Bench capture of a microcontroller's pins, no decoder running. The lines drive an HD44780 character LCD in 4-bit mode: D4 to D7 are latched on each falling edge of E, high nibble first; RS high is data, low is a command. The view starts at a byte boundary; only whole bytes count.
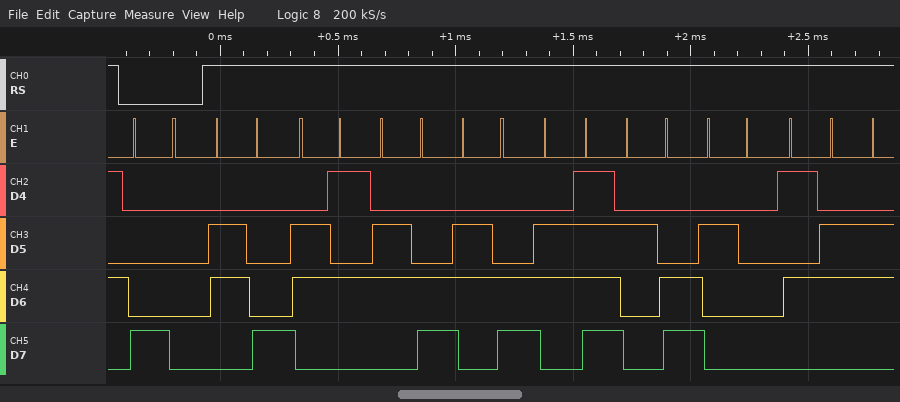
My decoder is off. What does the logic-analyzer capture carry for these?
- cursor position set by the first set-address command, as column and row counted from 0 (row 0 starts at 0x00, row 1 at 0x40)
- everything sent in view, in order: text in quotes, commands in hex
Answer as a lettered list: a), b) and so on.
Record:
a) column 0, row 0
b) 0x80 "hello, V"
